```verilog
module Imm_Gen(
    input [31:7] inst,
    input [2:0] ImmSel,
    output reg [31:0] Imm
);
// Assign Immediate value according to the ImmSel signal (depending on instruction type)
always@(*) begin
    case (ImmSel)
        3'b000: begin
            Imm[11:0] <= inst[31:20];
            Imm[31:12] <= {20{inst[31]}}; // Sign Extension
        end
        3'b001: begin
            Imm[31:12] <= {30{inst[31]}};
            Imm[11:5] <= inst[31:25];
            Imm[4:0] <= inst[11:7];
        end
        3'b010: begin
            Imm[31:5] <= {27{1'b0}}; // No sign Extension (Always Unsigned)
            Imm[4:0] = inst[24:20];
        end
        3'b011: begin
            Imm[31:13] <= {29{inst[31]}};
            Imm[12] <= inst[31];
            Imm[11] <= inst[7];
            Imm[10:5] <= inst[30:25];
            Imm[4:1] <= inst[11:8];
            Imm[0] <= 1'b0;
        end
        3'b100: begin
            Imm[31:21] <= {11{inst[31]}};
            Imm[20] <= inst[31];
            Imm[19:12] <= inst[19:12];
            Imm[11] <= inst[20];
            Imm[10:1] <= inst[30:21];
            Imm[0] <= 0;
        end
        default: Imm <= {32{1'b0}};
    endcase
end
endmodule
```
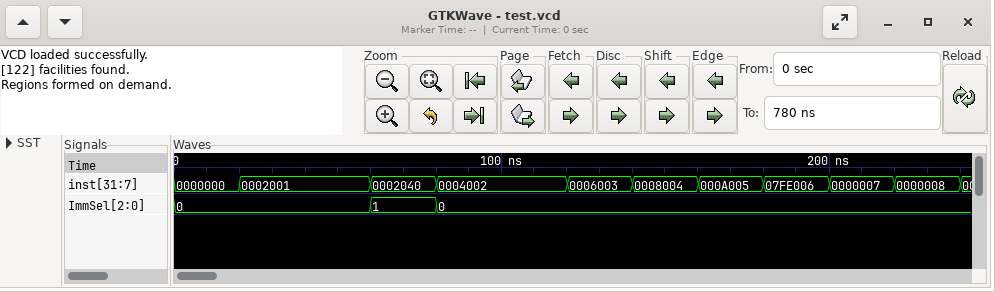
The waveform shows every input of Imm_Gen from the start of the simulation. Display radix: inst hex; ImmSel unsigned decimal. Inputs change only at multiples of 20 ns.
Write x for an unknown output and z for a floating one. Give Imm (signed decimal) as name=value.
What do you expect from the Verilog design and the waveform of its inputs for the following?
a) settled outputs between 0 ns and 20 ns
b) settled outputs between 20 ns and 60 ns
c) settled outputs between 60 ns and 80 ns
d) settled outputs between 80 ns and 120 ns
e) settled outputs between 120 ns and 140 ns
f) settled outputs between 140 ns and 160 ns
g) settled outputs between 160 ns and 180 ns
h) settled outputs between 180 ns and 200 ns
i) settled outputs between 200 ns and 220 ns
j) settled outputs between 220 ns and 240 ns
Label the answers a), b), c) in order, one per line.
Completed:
a) Imm=0
b) Imm=1
c) Imm=0
d) Imm=2
e) Imm=3
f) Imm=4
g) Imm=5
h) Imm=1023
i) Imm=0
j) Imm=0
